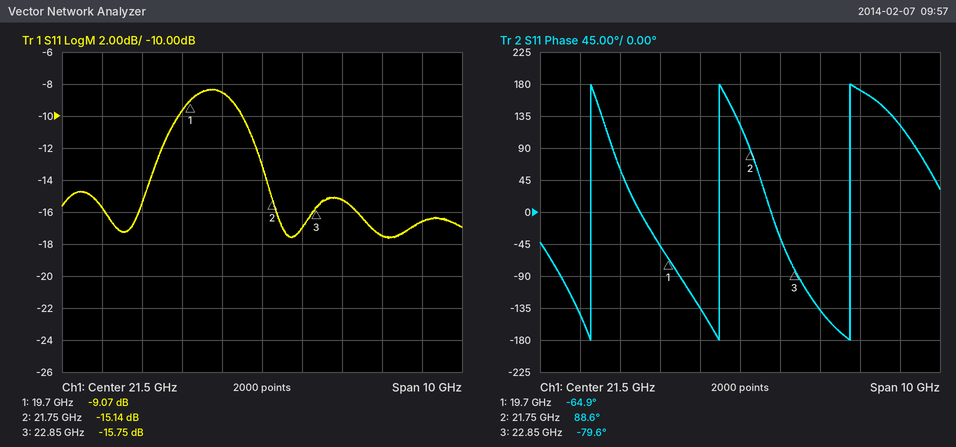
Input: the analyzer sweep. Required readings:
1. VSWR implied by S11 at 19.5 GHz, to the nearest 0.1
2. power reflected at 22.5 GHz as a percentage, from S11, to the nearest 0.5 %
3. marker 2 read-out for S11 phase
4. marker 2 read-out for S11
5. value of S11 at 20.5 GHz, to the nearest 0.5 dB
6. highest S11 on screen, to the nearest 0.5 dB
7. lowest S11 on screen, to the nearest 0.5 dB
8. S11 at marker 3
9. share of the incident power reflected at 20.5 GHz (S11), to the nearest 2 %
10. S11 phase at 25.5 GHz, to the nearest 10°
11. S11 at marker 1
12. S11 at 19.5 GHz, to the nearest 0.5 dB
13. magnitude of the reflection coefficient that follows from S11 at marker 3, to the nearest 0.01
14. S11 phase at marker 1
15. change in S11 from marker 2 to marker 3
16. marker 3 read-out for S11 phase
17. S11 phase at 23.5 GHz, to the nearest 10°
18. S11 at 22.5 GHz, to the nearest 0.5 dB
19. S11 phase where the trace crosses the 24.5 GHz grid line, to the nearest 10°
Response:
2.0
2.0 %
88.6°
-15.14 dB
-8.5 dB
-8.5 dB
-17.5 dB
-15.75 dB
14 %
120°
-9.07 dB
-9.5 dB
0.16
-64.9°
-0.61 dB
-79.6°
-140°
-17.0 dB
170°
